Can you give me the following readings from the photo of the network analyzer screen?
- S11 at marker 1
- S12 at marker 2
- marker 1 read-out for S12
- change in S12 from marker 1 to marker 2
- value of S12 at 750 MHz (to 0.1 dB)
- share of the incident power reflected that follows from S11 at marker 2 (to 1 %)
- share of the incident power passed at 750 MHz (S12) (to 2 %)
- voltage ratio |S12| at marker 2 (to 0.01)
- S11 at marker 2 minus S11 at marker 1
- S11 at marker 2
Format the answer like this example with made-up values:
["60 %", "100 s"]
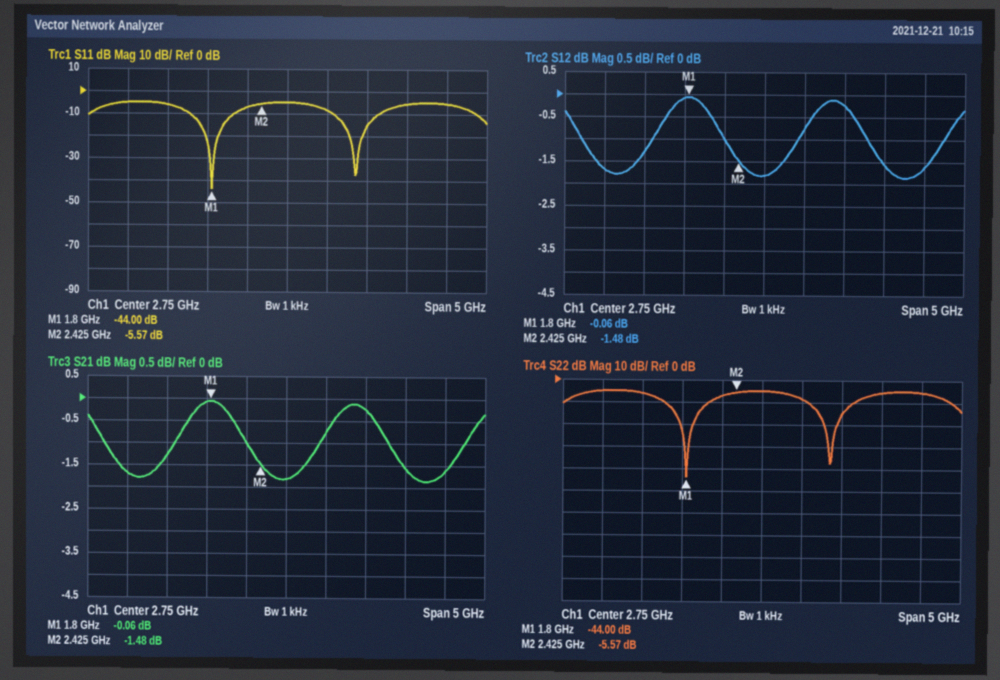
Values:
["-44.00 dB", "-1.48 dB", "-0.06 dB", "-1.42 dB", "-1.7 dB", "28 %", "68 %", "0.84", "38.43 dB", "-5.57 dB"]
